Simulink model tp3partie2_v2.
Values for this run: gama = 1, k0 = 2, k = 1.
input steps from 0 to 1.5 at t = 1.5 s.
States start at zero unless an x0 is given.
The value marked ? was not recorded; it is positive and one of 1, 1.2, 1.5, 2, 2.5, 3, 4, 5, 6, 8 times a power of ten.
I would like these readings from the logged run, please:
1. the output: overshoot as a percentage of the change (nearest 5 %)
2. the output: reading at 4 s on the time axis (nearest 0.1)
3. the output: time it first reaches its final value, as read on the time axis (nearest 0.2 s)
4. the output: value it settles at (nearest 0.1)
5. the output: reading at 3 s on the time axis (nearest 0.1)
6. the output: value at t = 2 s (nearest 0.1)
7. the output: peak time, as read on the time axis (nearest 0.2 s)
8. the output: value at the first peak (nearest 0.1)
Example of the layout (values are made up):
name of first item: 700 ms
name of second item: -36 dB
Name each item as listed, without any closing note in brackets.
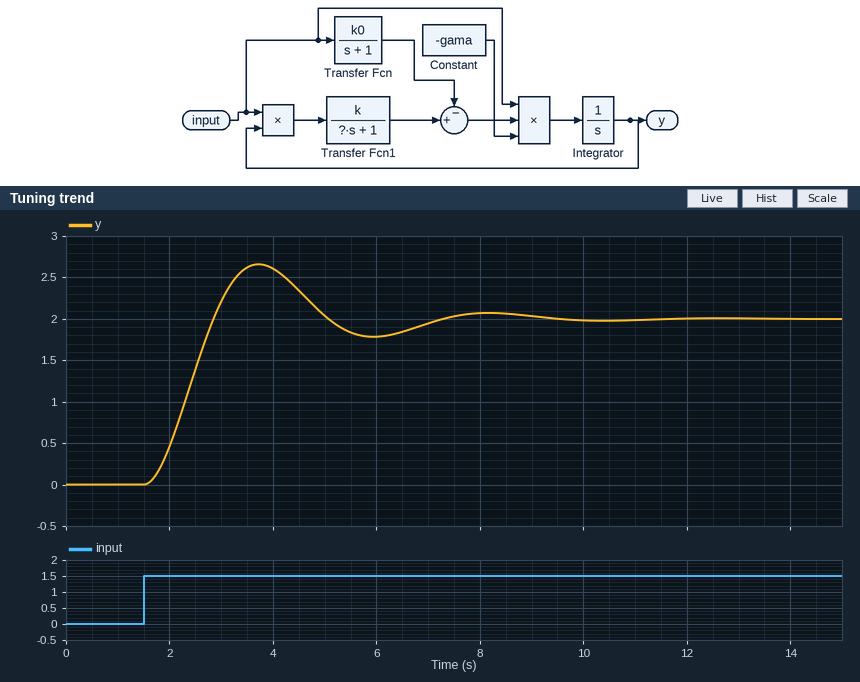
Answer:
the output: overshoot as a percentage of the change: 35 %
the output: reading at 4 s on the time axis: 2.6
the output: time it first reaches its final value, as read on the time axis: 2.8 s
the output: value it settles at: 2.0
the output: reading at 3 s on the time axis: 2.2
the output: value at t = 2 s: 0.5
the output: peak time, as read on the time axis: 3.8 s
the output: value at the first peak: 2.7
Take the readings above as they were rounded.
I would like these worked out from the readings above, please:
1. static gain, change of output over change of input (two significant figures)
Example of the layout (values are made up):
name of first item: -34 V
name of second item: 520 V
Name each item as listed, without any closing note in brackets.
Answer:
static gain, change of output over change of input: 1.3
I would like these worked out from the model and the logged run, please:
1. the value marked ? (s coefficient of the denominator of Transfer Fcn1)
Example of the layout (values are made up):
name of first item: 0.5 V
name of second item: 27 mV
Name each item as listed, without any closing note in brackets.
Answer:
the value marked ?: 1
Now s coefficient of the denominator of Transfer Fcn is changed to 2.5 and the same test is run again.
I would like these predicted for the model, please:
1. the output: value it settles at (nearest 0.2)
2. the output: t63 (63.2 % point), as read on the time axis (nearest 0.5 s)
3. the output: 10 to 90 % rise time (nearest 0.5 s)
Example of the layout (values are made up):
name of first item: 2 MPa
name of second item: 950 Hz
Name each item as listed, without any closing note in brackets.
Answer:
the output: value it settles at: 2.0
the output: t63 (63.2 % point), as read on the time axis: 3.0 s
the output: 10 to 90 % rise time: 5.0 s
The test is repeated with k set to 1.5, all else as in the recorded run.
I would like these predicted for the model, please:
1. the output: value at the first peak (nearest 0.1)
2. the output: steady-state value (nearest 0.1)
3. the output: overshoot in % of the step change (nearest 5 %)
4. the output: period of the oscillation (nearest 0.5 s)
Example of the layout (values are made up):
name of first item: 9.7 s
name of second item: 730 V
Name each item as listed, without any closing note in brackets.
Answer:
the output: value at the first peak: 1.9
the output: steady-state value: 1.3
the output: overshoot in % of the step change: 40 %
the output: period of the oscillation: 3.5 s
